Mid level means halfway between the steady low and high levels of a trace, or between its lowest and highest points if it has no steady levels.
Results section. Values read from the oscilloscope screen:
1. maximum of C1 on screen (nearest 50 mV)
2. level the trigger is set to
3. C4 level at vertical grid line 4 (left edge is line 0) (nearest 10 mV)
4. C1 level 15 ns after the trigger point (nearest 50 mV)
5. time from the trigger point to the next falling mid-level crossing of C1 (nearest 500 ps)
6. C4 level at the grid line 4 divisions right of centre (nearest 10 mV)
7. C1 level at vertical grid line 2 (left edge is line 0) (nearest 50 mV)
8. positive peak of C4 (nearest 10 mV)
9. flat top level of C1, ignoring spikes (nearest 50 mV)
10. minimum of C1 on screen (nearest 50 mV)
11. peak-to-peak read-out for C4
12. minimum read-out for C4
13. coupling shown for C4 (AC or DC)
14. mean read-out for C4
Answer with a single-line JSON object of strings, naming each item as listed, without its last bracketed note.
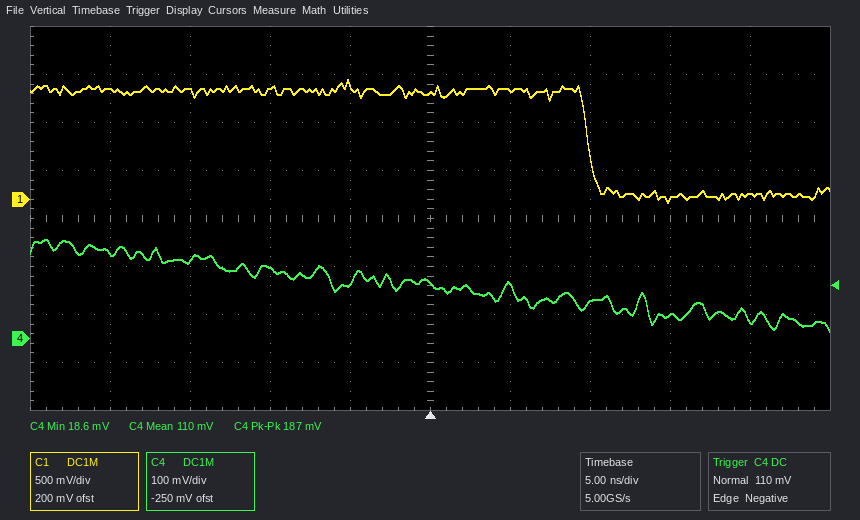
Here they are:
{"maximum of C1 on screen": "1.25 V", "level the trigger is set to": "110 mV", "C4 level at vertical grid line 4 (left edge is line 0)": "120 mV", "C1 level 15 ns after the trigger point": "0 mV", "time from the trigger point to the next falling mid-level crossing of C1": "10.0 ns", "C4 level at the grid line 4 divisions right of centre": "40 mV", "C1 level at vertical grid line 2 (left edge is line 0)": "1.10 V", "positive peak of C4": "210 mV", "flat top level of C1, ignoring spikes": "1.15 V", "minimum of C1 on screen": "-50 mV", "peak-to-peak read-out for C4": "187 mV", "minimum read-out for C4": "18.6 mV", "coupling shown for C4": "DC", "mean read-out for C4": "110 mV"}
